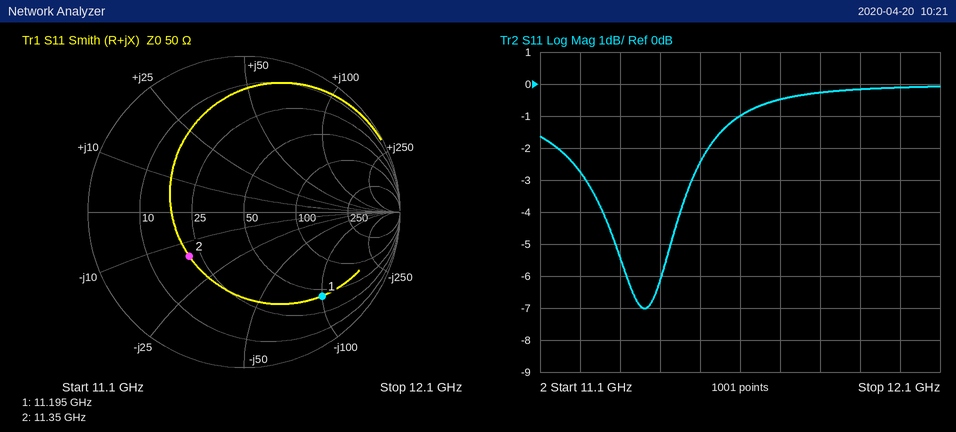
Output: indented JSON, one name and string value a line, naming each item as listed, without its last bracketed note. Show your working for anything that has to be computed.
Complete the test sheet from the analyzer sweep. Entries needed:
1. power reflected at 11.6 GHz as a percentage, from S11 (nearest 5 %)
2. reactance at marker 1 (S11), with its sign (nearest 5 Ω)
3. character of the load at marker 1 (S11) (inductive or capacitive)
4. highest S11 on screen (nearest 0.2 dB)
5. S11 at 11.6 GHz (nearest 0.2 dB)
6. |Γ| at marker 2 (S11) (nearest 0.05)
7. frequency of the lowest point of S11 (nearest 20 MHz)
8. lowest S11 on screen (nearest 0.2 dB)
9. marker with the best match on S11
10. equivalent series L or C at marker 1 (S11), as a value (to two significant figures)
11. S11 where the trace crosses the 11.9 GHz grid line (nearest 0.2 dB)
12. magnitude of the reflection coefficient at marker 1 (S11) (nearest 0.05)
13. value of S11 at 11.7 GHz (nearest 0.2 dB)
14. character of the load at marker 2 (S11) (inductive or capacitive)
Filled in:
{
  "power reflected at 11.6 GHz as a percentage, from S11": "10^(-1/10) ≈ 79.4 %, so 80 % to the nearest 5 %",
  "reactance at marker 1 (S11), with its sign": "-100 Ω",
  "character of the load at marker 1 (S11)": "capacitive",
  "highest S11 on screen": "0.0 dB",
  "S11 at 11.6 GHz": "-1.0 dB",
  "|Γ| at marker 2 (S11)": "0.45",
  "frequency of the lowest point of S11": "11.36 GHz",
  "lowest S11 on screen": "-7.0 dB",
  "marker with the best match on S11": "marker 2",
  "equivalent series L or C at marker 1 (S11), as a value": "C = 1/(2π × 11.195 GHz × 100 Ω) ≈ 142 fF, so 140 fF to two significant figures",
  "S11 where the trace crosses the 11.9 GHz grid line": "-0.2 dB",
  "magnitude of the reflection coefficient at marker 1 (S11)": "0.75",
  "value of S11 at 11.7 GHz": "-0.4 dB",
  "character of the load at marker 2 (S11)": "capacitive"
}
